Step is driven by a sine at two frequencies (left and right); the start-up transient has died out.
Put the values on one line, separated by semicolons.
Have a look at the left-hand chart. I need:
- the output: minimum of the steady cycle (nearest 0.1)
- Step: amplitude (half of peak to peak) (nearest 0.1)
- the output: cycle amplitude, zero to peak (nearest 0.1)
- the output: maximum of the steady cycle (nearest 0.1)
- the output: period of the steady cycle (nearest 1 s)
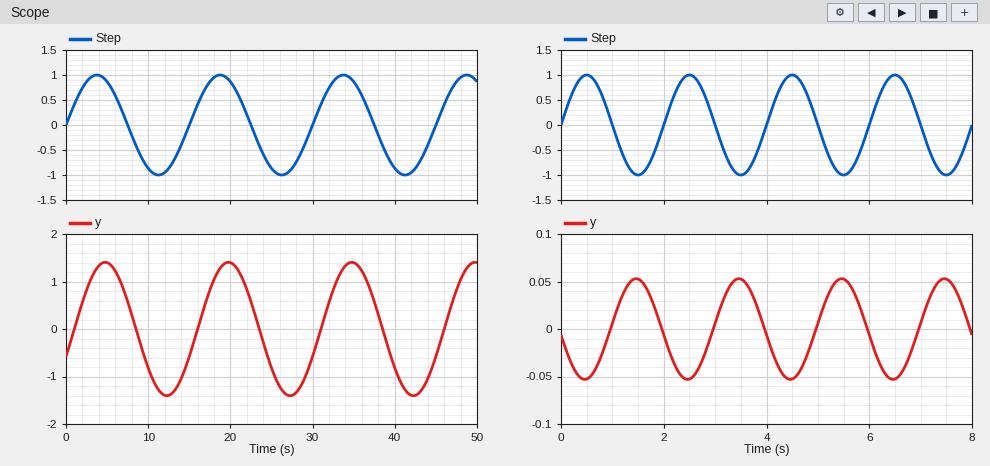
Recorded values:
-1.4; 1.0; 1.4; 1.4; 15 s
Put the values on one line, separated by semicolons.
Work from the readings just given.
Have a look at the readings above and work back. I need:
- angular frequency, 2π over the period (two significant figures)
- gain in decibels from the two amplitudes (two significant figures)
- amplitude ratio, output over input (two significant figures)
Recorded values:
0.42 rad/s; 2.9 dB; 1.4
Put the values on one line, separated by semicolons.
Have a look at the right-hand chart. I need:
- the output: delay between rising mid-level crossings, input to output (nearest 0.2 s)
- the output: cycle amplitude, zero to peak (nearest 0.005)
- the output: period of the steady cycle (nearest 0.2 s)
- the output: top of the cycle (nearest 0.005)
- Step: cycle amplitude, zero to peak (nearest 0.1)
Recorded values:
1.0 s; 0.055; 2.0 s; 0.055; 1.0
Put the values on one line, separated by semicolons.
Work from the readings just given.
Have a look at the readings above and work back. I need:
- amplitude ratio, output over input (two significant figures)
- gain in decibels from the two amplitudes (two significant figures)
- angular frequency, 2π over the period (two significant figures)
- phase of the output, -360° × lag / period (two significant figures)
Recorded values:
0.055; -25 dB; 3.1 rad/s; -180°
